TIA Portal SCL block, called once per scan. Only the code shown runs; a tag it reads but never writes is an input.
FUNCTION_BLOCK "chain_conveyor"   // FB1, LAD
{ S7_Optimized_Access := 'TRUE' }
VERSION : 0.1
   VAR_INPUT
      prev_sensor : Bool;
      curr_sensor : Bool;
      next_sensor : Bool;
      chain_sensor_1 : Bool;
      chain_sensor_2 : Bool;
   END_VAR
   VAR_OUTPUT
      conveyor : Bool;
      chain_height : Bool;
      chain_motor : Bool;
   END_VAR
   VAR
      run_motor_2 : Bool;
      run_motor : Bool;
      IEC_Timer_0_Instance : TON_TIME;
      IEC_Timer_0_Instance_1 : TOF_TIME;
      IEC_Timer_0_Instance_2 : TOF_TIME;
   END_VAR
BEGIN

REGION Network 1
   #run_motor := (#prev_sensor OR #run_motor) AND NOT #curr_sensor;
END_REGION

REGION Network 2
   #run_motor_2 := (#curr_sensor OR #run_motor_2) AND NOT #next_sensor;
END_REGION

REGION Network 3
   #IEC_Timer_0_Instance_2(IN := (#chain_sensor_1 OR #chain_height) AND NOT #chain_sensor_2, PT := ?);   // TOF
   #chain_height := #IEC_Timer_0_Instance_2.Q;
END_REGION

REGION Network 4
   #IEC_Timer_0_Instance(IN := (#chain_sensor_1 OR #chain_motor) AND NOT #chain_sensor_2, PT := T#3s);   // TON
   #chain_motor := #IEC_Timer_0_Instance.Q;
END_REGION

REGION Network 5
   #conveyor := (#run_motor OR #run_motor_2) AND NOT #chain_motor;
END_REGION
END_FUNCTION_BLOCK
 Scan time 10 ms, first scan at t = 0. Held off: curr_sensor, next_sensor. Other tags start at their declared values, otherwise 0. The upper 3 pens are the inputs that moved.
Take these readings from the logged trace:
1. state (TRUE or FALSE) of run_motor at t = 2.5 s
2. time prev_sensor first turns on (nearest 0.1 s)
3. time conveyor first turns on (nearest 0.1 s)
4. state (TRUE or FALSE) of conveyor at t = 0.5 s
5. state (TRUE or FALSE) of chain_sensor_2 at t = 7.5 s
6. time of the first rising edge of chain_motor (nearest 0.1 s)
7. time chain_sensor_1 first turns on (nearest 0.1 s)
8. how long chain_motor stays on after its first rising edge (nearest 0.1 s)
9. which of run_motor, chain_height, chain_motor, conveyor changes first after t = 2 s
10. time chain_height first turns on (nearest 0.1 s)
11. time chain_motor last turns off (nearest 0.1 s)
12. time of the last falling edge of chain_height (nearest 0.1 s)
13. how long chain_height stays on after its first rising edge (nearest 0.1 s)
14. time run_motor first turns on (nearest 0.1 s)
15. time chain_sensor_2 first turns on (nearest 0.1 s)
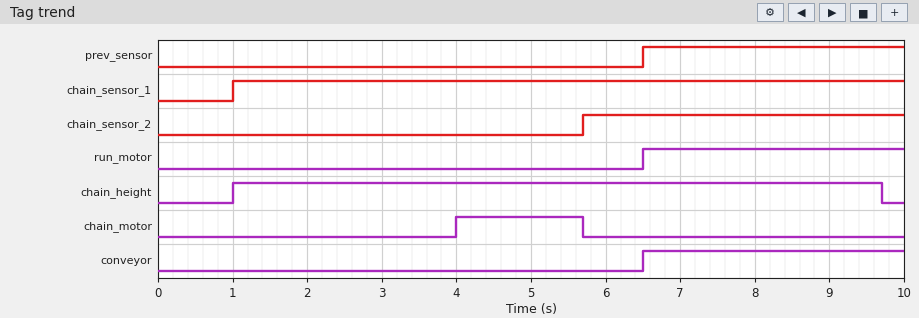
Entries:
FALSE
6.5 s
6.5 s
FALSE
TRUE
4.0 s
1.0 s
1.7 s
chain_motor
1.0 s
5.7 s
9.7 s
8.7 s
6.5 s
5.7 s
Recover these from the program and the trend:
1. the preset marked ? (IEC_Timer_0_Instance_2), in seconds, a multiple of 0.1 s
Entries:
4.0 s
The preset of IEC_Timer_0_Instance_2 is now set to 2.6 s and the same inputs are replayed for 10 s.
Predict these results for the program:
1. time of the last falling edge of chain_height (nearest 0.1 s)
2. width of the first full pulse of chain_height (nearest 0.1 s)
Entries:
8.3 s
7.3 s
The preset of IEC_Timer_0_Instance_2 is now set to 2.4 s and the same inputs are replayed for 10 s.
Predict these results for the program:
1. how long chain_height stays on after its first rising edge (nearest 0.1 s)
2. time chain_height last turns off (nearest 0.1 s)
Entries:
7.1 s
8.1 s
